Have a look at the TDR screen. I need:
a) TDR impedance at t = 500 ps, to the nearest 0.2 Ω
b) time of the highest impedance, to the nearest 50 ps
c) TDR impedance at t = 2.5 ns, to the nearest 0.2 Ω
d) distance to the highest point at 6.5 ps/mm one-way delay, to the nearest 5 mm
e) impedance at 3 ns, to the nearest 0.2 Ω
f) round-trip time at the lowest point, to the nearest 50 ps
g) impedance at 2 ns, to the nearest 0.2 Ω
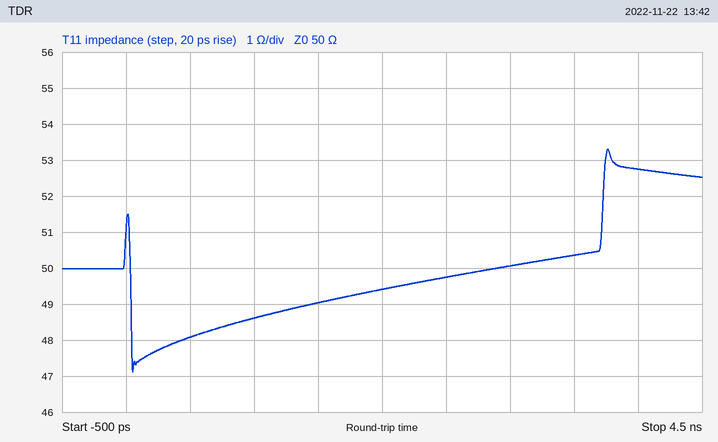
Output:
48.0 Ω
3.75 ns
49.8 Ω
290 mm
50.0 Ω
50 ps
49.4 Ω
